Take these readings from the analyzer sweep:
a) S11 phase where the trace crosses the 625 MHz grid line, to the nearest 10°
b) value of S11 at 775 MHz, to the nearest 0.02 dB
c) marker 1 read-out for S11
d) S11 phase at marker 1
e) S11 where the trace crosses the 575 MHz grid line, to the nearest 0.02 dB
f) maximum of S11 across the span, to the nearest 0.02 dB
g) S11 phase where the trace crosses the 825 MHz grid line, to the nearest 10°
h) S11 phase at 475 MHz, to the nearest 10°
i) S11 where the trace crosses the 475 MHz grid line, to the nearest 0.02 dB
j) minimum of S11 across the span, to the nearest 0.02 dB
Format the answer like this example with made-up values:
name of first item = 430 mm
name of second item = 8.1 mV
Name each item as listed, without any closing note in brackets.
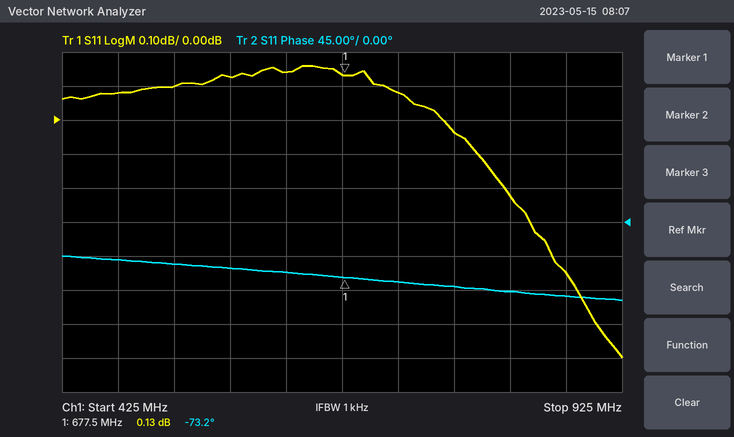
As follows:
S11 phase where the trace crosses the 625 MHz grid line, to the nearest 10° = -70°
value of S11 at 775 MHz, to the nearest 0.02 dB = -0.04 dB
marker 1 read-out for S11 = 0.13 dB
S11 phase at marker 1 = -73.2°
S11 where the trace crosses the 575 MHz grid line, to the nearest 0.02 dB = 0.12 dB
maximum of S11 across the span, to the nearest 0.02 dB = 0.16 dB
S11 phase where the trace crosses the 825 MHz grid line, to the nearest 10° = -90°
S11 phase at 475 MHz, to the nearest 10° = -50°
S11 where the trace crosses the 475 MHz grid line, to the nearest 0.02 dB = 0.08 dB
minimum of S11 across the span, to the nearest 0.02 dB = -0.70 dB
